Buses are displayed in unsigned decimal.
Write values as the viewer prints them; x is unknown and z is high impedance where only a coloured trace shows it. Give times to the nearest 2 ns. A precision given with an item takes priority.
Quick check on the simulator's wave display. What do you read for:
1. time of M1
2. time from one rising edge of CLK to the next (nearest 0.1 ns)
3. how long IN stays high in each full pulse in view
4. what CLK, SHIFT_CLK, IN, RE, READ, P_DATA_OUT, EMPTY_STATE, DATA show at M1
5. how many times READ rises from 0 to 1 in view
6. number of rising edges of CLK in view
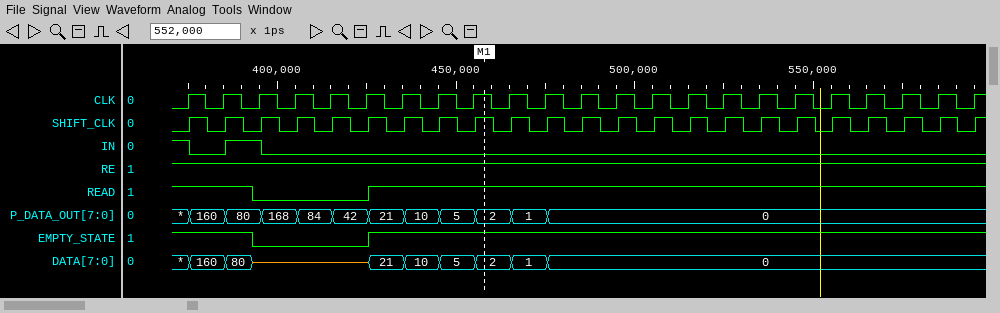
458 ns
10 ns
10 ns
CLK=1, SHIFT_CLK=1, IN=0, RE=1, READ=1, P_DATA_OUT=2, EMPTY_STATE=1, DATA=2
1
23
